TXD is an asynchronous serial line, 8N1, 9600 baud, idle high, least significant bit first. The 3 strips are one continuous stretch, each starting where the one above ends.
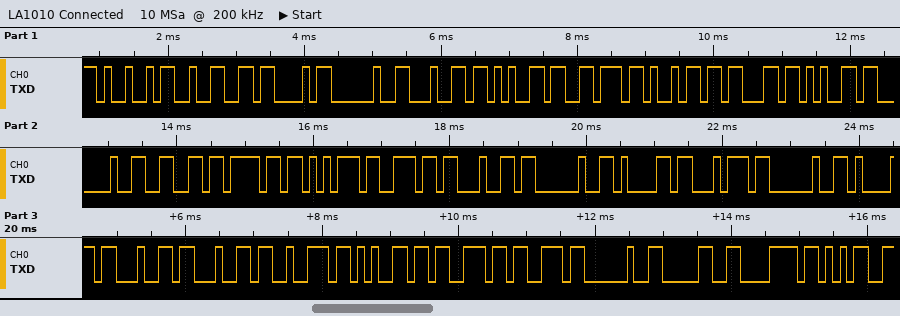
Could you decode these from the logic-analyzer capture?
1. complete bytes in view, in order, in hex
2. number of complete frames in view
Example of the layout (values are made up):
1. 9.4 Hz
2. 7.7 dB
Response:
1. 49 32 43 20 64 65 76 69 63 65 20 66 6F 75 6E 64 20 61 74 20 61 64 64 72 65 73 73 20 30 78 35
2. 31
